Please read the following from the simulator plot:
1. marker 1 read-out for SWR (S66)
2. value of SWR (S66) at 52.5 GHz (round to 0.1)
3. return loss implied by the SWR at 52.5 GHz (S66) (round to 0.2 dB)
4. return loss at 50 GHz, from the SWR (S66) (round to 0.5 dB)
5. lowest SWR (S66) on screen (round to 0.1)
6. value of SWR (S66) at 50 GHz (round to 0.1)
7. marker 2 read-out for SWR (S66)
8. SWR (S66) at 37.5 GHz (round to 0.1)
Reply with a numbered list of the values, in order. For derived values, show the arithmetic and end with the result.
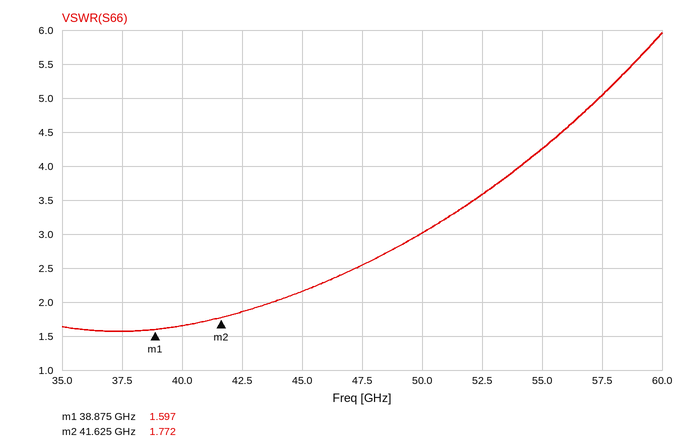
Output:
1. 1.597
2. 3.6
3. −20 log10((3.6 − 1)/(3.6 + 1)) ≈ 5.0 dB
4. −20 log10((3 − 1)/(3 + 1)) ≈ 6.0 dB
5. 1.6
6. 3.0
7. 1.772
8. 1.6
